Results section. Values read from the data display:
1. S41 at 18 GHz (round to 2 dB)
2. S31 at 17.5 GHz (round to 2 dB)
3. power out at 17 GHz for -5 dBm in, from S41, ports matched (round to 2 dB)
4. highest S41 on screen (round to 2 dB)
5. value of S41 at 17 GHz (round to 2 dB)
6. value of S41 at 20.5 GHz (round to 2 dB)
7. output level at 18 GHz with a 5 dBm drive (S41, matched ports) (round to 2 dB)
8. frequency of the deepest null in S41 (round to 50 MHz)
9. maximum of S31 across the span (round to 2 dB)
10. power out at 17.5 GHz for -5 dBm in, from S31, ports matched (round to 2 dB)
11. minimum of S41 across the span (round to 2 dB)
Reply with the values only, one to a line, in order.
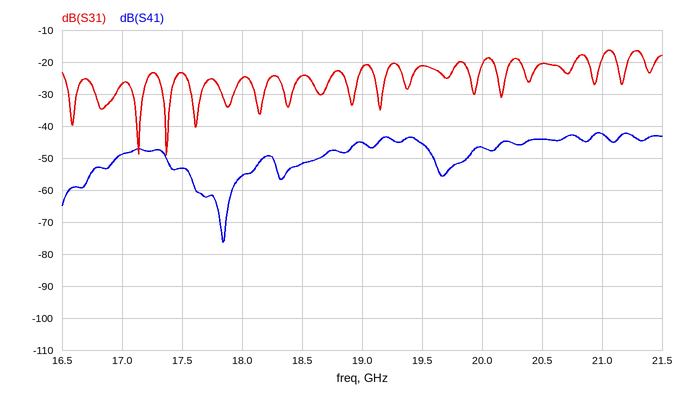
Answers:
-56 dB
-24 dB
-54 dBm
-42 dB
-48 dB
-44 dB
-50 dBm
17.85 GHz
-16 dB
-28 dBm
-76 dB
